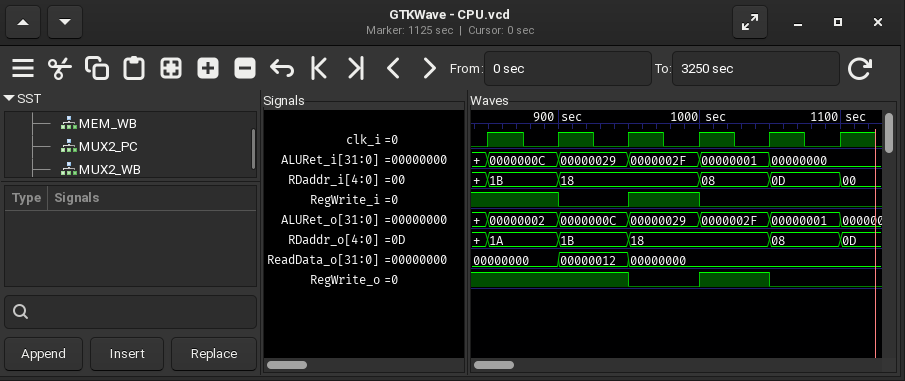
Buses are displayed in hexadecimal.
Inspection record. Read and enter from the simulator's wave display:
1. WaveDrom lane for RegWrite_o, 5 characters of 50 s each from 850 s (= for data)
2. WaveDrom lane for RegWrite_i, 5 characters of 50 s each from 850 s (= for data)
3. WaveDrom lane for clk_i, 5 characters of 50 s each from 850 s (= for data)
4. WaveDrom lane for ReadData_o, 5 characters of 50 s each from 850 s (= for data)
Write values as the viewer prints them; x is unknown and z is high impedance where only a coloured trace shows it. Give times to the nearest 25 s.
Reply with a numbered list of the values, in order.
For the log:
1. {name: 'RegWrite_o', wave: '1.010'}
2. {name: 'RegWrite_i', wave: '1010.'}
3. {name: 'clk_i', wave: 'p....'}
4. {name: 'ReadData_o', wave: '===..', data: '00000000 00000012 00000000'}
